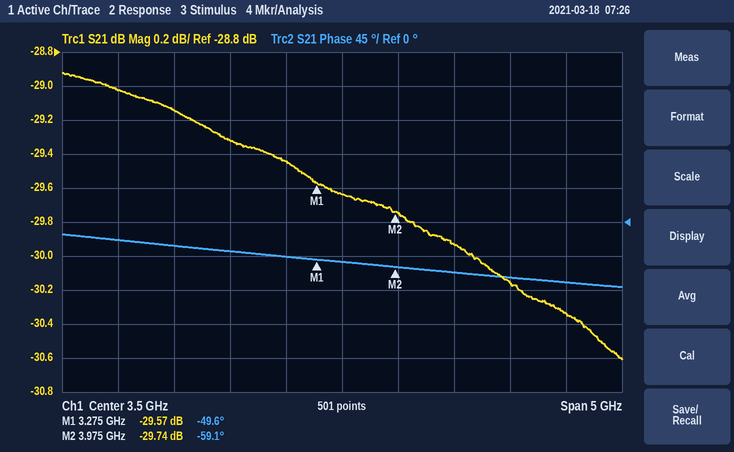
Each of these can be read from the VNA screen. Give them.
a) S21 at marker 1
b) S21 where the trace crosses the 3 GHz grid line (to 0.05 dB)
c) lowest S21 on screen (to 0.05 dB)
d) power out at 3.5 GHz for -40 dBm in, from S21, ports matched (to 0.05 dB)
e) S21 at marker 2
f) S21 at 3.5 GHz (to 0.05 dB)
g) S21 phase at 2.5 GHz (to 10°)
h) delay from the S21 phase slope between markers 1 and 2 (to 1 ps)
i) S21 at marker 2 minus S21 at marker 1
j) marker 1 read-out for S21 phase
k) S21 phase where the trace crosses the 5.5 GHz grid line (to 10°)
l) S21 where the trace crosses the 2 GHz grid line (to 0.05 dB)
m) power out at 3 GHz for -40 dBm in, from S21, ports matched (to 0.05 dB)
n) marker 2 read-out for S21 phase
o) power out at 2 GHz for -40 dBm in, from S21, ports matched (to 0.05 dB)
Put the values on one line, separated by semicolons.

-29.57 dB; -29.45 dB; -30.60 dB; -69.65 dBm; -29.74 dB; -29.65 dB; -40°; 38 ps; -0.17 dB; -49.6°; -80°; -29.15 dB; -69.45 dBm; -59.1°; -69.15 dBm
